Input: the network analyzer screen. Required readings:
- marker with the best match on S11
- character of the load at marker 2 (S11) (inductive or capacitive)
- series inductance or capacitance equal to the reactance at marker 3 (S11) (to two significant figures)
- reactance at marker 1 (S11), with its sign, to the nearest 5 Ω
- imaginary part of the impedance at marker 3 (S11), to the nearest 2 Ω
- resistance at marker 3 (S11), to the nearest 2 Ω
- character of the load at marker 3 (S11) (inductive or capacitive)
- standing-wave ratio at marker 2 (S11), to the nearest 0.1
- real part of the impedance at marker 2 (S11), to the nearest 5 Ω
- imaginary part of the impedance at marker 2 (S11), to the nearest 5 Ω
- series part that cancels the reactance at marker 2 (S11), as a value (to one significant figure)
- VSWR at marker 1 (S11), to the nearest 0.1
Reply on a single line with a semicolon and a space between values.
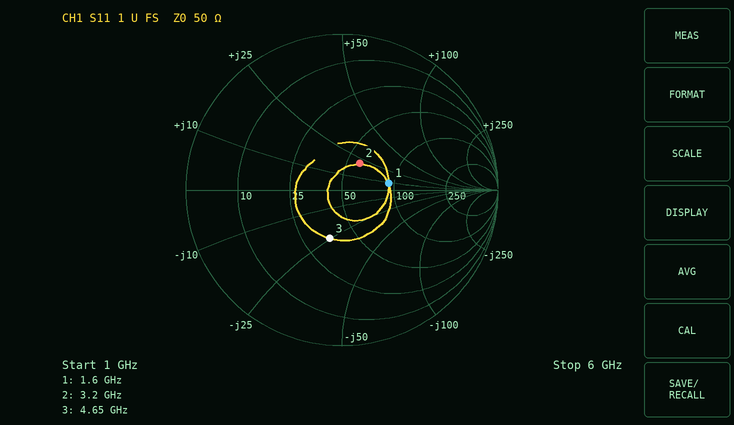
marker 2; inductive; 1.4 pF; +10 Ω; -24 Ω; 36 Ω; capacitive; 1.5; 60 Ω; +20 Ω; 2 pF; 1.9
